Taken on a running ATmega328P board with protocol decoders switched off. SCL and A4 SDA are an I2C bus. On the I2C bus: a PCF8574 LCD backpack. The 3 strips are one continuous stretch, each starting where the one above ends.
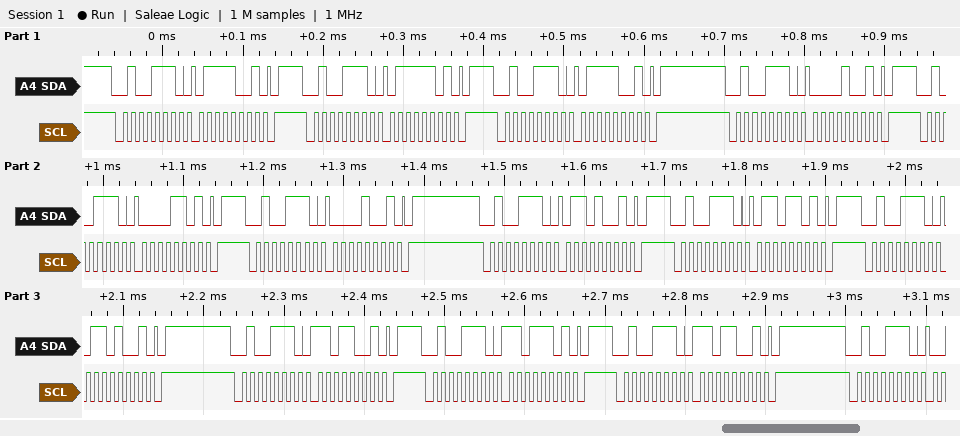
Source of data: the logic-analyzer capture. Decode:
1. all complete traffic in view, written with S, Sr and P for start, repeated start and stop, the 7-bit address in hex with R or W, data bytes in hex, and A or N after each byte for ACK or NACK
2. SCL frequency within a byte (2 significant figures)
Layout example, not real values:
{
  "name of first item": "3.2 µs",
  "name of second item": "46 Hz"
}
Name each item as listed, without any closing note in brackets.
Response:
{
  "all complete traffic in view, written with S, Sr and P for start, repeated start and stop, the 7-bit address in hex with R or W, data bytes in hex, and A or N after each byte for ACK or NACK": "S 27W A 79 A P S 27W A 7D A P S 27W A 79 A P S 27W A 09 A P S 27W A 0D A P S 27W A 09 A P S 27W A 69 A P S 27W A 6D A P S 27W A 69 A P S 27W A D9 A P S 27W A DD A P S 27W A D9 A P S 27W A",
  "SCL frequency within a byte": "100 kHz"
}
